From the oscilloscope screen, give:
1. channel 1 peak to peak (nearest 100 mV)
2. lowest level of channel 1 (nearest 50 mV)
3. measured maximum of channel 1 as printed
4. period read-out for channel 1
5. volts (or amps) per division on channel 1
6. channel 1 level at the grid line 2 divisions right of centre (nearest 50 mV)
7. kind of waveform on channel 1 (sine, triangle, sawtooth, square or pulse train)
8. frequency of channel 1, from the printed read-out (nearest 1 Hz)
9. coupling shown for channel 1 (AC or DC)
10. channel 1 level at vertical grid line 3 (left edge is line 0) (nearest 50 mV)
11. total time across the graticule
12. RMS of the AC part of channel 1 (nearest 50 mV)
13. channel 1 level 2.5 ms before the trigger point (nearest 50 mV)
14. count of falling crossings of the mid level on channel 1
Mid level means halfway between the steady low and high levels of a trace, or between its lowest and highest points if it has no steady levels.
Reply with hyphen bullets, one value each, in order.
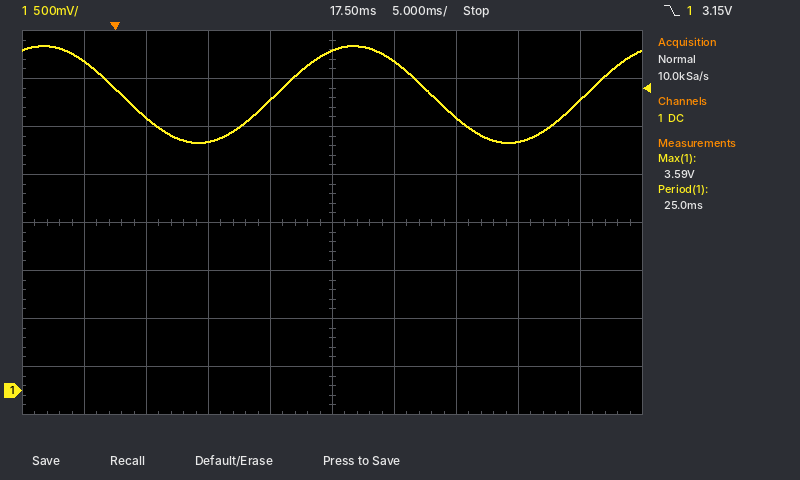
- 1.00 V
- 2.60 V
- 3.59 V
- 25.0 ms
- 500 mV
- 2.85 V
- sine
- 40 Hz
- DC
- 2.60 V
- 50 ms
- 350 mV
- 3.45 V
- 2
